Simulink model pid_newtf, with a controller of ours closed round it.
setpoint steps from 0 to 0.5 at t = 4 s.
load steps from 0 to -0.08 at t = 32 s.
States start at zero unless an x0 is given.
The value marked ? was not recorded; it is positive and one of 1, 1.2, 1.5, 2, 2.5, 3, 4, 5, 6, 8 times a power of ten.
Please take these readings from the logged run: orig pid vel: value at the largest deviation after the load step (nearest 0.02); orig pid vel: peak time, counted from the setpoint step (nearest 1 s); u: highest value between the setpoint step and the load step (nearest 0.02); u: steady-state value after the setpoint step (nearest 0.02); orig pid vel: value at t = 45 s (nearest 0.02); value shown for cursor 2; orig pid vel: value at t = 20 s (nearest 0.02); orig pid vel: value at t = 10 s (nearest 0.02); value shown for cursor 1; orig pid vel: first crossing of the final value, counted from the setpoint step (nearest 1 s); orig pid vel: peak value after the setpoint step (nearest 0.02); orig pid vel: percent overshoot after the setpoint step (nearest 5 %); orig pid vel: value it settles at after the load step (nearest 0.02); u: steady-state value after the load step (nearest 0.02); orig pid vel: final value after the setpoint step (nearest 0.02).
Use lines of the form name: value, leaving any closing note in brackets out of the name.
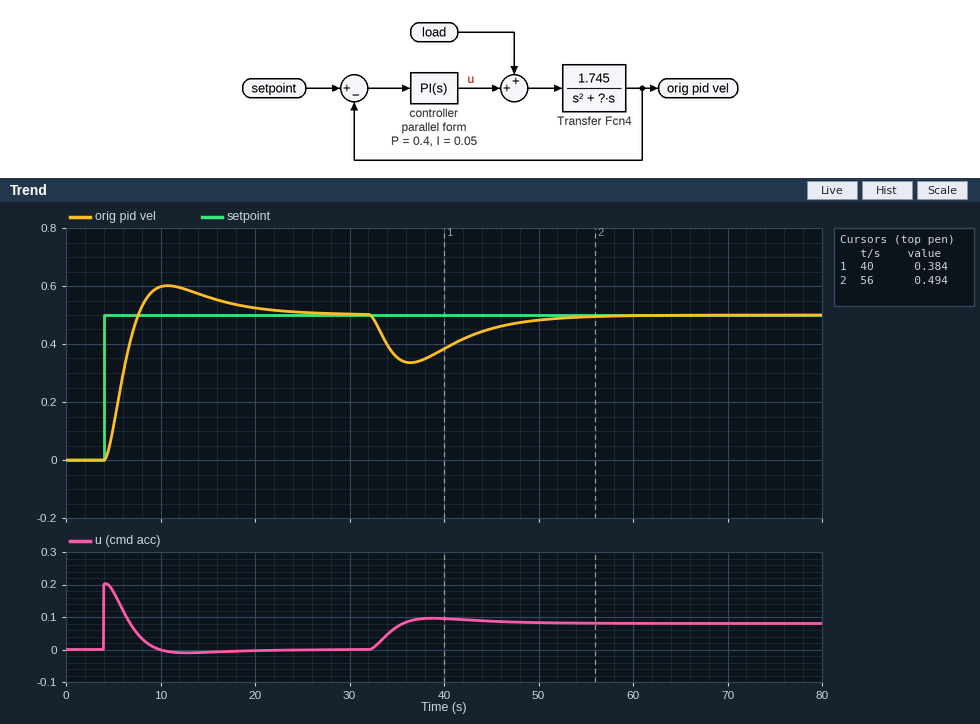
orig pid vel: value at the largest deviation after the load step: 0.34
orig pid vel: peak time, counted from the setpoint step: 7 s
u: highest value between the setpoint step and the load step: 0.20
u: steady-state value after the setpoint step: 0.00
orig pid vel: value at t = 45 s: 0.46
value shown for cursor 2: 0.494
orig pid vel: value at t = 20 s: 0.52
orig pid vel: value at t = 10 s: 0.60
value shown for cursor 1: 0.384
orig pid vel: first crossing of the final value, counted from the setpoint step: 4 s
orig pid vel: peak value after the setpoint step: 0.60
orig pid vel: percent overshoot after the setpoint step: 20 %
orig pid vel: value it settles at after the load step: 0.50
u: steady-state value after the load step: 0.08
orig pid vel: final value after the setpoint step: 0.50
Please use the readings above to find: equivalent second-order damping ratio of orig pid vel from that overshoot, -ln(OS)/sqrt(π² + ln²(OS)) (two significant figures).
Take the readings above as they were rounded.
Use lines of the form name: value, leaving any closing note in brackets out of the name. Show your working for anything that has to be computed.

equivalent second-order damping ratio of orig pid vel from that overshoot, -ln(OS)/sqrt(π² + ln²(OS)): ln(0.2) = -1.609; 1.609 / sqrt(9.870 + 2.590) = 0.46
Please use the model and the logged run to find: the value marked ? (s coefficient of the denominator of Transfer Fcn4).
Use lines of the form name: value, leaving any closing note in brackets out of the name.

the value marked ?: 1.5
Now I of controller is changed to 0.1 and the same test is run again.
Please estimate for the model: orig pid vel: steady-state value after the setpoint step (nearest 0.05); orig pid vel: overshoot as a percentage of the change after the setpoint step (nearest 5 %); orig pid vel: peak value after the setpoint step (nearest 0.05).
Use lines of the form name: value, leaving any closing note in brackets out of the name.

orig pid vel: steady-state value after the setpoint step: 0.50
orig pid vel: overshoot as a percentage of the change after the setpoint step: 35 %
orig pid vel: peak value after the setpoint step: 0.65
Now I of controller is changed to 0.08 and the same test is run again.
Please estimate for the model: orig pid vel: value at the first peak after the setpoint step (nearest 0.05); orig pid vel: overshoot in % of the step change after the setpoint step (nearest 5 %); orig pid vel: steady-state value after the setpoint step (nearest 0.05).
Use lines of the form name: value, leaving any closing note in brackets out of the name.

orig pid vel: value at the first peak after the setpoint step: 0.65
orig pid vel: overshoot in % of the step change after the setpoint step: 30 %
orig pid vel: steady-state value after the setpoint step: 0.50
